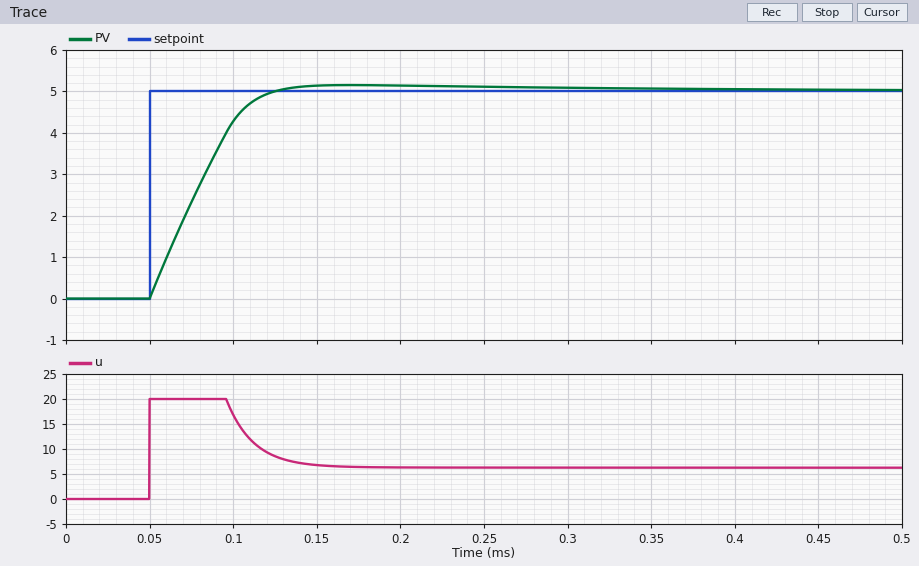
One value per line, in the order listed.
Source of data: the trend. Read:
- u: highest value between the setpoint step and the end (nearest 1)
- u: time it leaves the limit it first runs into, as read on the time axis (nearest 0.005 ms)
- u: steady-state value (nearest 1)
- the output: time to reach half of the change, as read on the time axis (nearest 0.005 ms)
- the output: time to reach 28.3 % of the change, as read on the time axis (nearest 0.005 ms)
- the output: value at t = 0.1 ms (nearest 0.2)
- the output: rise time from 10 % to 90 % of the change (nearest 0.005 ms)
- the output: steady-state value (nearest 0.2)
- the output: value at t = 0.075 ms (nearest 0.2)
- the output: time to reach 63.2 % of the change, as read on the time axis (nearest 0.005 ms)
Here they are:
20
0.095 ms
6
0.075 ms
0.065 ms
4.2
0.050 ms
5.0
2.4
0.085 ms
